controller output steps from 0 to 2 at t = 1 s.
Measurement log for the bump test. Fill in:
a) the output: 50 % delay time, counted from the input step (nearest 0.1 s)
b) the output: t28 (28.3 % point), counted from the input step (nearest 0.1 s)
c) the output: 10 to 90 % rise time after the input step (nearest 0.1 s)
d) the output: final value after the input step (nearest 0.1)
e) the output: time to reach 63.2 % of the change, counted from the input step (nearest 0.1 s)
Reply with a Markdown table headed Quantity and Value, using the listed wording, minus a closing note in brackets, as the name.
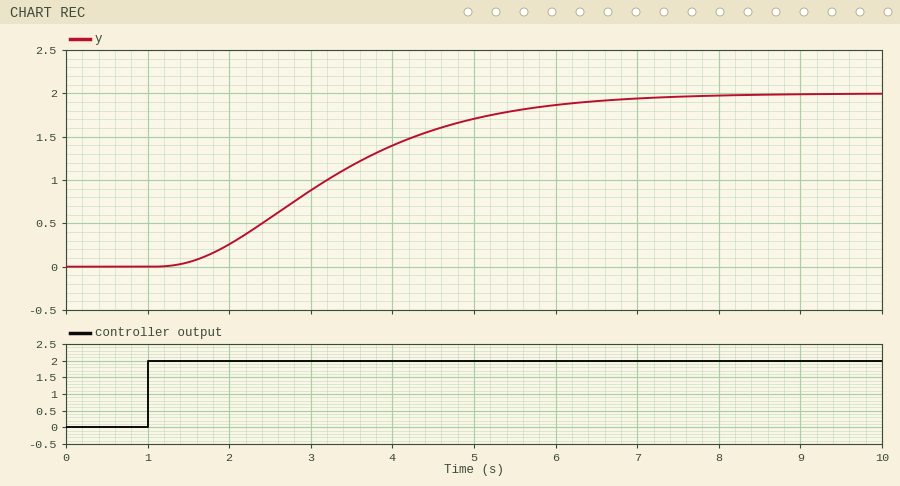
| Quantity | Value |
|---|---|
| the output: 50 % delay time, counted from the input step | 2.2 s |
| the output: t28 (28.3 % point), counted from the input step | 1.5 s |
| the output: 10 to 90 % rise time after the input step | 3.6 s |
| the output: final value after the input step | 2.0 |
| the output: time to reach 63.2 % of the change, counted from the input step | 2.7 s |
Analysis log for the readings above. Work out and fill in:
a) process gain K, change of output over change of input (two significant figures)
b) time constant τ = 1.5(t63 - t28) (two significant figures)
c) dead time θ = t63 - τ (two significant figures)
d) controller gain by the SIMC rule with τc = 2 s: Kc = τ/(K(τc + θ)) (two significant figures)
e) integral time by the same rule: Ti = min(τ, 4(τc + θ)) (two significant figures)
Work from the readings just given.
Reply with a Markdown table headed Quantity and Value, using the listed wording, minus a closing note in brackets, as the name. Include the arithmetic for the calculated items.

| Quantity | Value |
|---|---|
| process gain K, change of output over change of input | (2 - 0) / 2 = 1.0 |
| time constant τ = 1.5(t63 - t28) | 1.5 × (2.7 - 1.5) = 1.8 s |
| dead time θ = t63 - τ | 2.7 - 1.8 = 0.90 s |
| controller gain by the SIMC rule with τc = 2 s: Kc = τ/(K(τc + θ)) | 1.8 / (1 × (2 + 0.9)) = 0.62 |
| integral time by the same rule: Ti = min(τ, 4(τc + θ)) | min(1.8, 4 × (2 + 0.9)) = 1.8 s |
